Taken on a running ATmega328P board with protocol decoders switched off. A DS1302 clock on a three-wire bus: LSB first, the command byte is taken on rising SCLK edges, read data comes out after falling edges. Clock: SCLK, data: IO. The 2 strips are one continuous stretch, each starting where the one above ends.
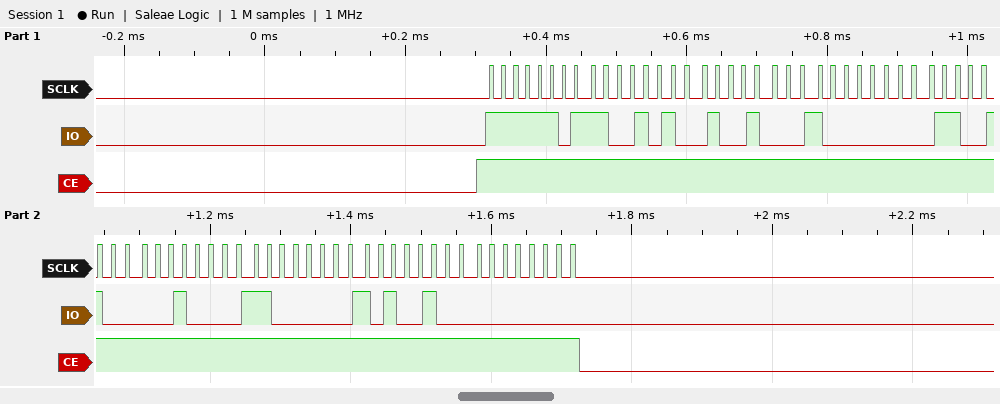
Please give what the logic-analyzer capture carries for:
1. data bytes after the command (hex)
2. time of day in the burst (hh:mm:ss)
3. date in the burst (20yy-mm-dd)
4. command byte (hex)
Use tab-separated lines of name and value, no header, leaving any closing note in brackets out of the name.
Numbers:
data bytes after the command	53 12 01 26 08 03 25 00
time of day in the burst	01:12:53
date in the burst	2025-08-26
command byte	0xBF
